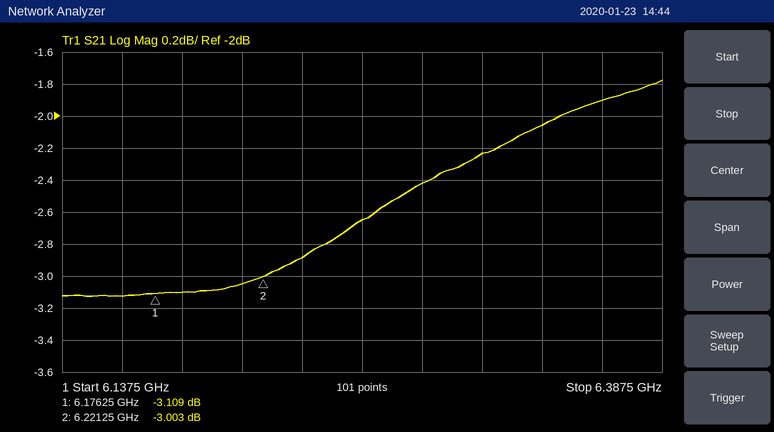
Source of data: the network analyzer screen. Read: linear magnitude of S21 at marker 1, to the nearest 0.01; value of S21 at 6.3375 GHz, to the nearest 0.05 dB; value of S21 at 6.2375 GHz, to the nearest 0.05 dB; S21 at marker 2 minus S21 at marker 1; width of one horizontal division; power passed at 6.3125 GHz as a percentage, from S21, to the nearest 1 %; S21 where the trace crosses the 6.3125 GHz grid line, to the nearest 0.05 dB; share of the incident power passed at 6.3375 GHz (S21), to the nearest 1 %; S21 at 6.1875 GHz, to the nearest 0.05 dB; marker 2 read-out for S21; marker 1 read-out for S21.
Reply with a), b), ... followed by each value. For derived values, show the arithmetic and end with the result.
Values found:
a) 10^(-3.109/20) ≈ 0.70
b) -2.05 dB
c) -2.90 dB
d) -3.003 − (-3.109) = 0.106 dB
e) 25 MHz
f) 10^(-2.25/10) ≈ 60 %
g) -2.25 dB
h) 10^(-2.05/10) ≈ 62 %
i) -3.10 dB
j) -3.003 dB
k) -3.109 dB
